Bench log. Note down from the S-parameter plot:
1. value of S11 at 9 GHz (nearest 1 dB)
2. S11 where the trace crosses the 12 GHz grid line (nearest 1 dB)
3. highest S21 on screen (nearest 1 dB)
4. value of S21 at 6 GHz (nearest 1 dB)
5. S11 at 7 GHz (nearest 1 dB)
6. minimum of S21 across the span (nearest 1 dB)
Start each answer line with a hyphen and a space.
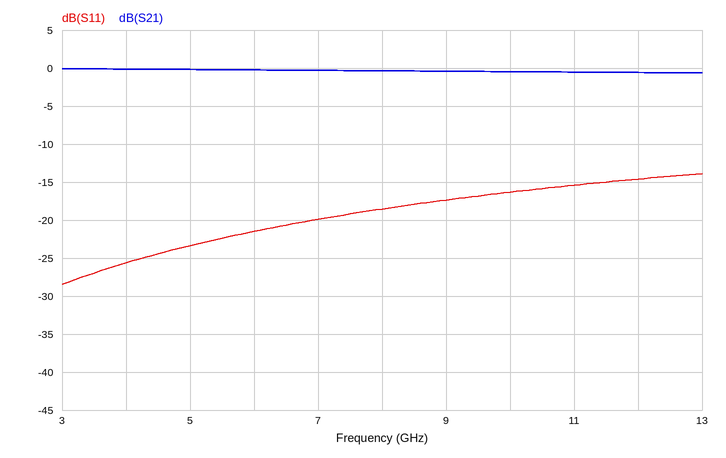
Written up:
- -17 dB
- -15 dB
- 0 dB
- 0 dB
- -20 dB
- -1 dB
